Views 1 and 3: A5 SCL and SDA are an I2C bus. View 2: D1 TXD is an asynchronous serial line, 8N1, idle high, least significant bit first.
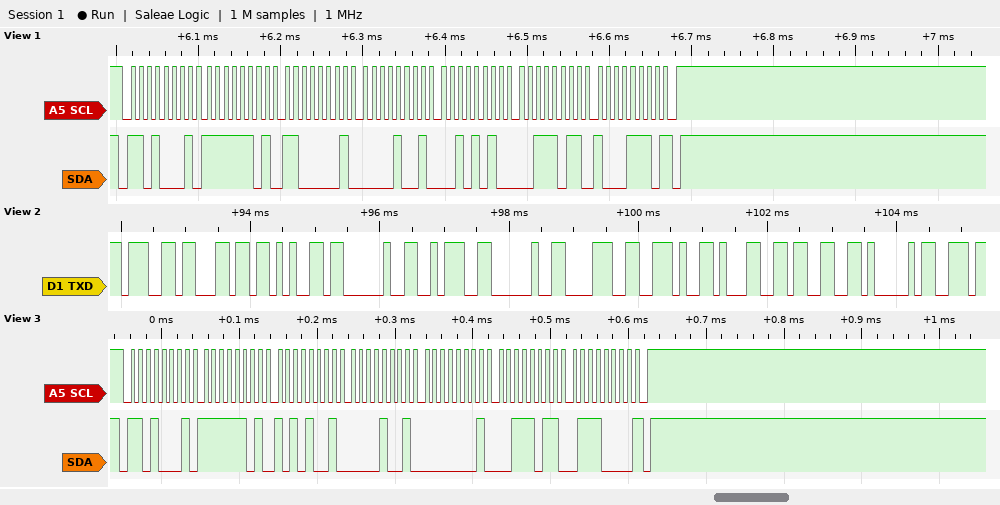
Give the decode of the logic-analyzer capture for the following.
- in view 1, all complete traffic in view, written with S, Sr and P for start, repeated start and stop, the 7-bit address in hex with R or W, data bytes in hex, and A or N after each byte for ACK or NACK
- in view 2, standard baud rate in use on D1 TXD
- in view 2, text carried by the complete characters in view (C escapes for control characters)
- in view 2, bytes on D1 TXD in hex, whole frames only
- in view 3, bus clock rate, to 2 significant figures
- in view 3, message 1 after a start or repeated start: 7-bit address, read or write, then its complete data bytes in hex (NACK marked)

S 68R A FD A C1 A 09 A 2A A 3B A 8E N P
9600 baud
"gle : 8.13A"
67 6C 65 20 3A 20 38 2E 31 33 41
100 kHz
0x68 read: FD A9 09 01 3B 70 NACK
